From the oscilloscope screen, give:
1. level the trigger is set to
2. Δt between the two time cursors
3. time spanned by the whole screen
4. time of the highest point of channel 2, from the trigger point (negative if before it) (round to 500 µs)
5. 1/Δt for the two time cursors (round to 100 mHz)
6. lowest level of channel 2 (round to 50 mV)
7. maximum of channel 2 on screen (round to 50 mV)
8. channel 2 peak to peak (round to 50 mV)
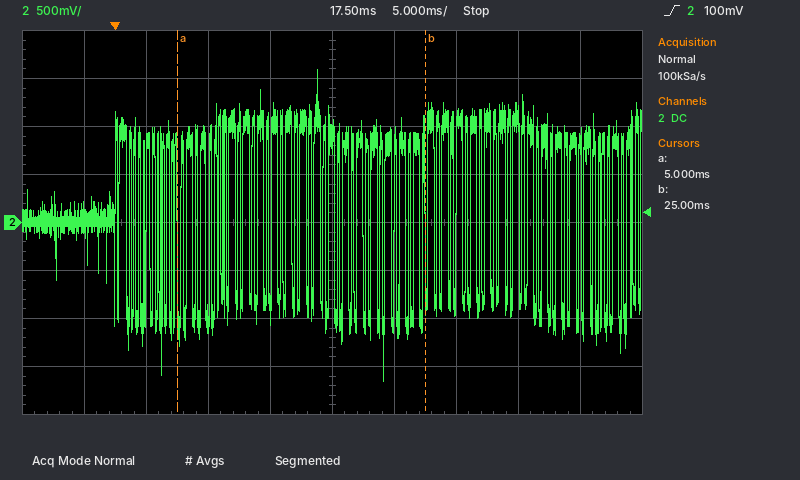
100 mV
20.0 ms
50 ms
+16.5 ms
50.0 Hz
-1.65 V
1.60 V
3.25 V
